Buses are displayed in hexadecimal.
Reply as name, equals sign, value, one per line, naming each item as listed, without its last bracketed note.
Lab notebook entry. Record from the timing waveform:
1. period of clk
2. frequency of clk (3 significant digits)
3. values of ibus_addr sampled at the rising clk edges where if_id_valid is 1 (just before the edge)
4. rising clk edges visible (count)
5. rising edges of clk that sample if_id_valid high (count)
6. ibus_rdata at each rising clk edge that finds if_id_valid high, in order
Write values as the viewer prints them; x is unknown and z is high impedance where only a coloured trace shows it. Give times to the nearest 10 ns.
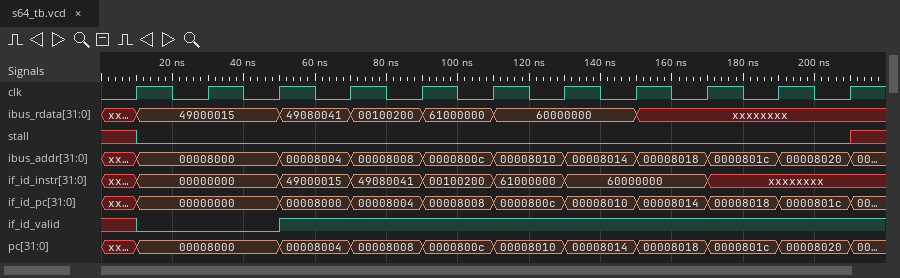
period of clk = 20 ns
frequency of clk = 50.0 MHz
values of ibus_addr sampled at the rising clk edges where if_id_valid is 1 = 00008004, 00008008, 0000800c, 00008010, 00008014, 00008018, 0000801c, 00008020
rising clk edges visible = 11
rising edges of clk that sample if_id_valid high = 8
ibus_rdata at each rising clk edge that finds if_id_valid high, in order = 49080041, 00100200, 61000000, 60000000, 60000000, xxxxxxxx, xxxxxxxx, xxxxxxxx
